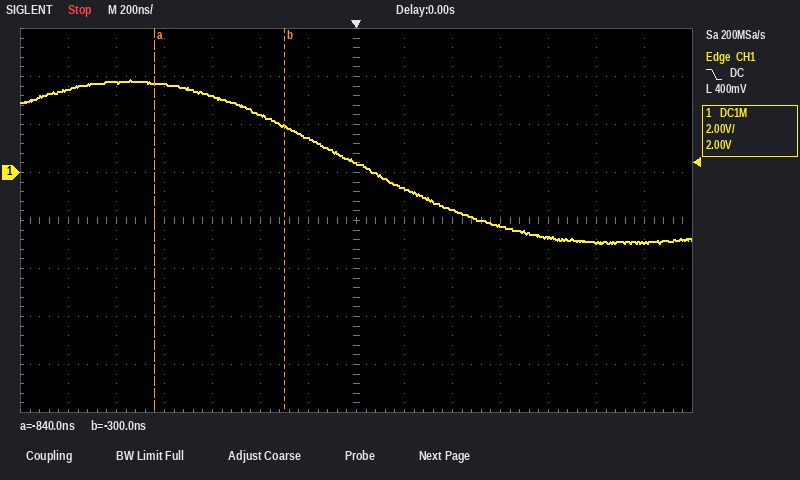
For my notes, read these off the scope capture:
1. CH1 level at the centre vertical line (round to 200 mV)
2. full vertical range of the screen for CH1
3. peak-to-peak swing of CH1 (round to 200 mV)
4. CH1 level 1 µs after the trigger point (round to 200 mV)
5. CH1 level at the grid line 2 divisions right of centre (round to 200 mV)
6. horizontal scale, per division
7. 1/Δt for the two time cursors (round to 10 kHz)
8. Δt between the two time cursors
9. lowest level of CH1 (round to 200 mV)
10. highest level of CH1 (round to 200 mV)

400 mV
16 V
6.8 V
-3.0 V
-1.6 V
200 ns
1.85 MHz
540 ns
-3.0 V
3.8 V
